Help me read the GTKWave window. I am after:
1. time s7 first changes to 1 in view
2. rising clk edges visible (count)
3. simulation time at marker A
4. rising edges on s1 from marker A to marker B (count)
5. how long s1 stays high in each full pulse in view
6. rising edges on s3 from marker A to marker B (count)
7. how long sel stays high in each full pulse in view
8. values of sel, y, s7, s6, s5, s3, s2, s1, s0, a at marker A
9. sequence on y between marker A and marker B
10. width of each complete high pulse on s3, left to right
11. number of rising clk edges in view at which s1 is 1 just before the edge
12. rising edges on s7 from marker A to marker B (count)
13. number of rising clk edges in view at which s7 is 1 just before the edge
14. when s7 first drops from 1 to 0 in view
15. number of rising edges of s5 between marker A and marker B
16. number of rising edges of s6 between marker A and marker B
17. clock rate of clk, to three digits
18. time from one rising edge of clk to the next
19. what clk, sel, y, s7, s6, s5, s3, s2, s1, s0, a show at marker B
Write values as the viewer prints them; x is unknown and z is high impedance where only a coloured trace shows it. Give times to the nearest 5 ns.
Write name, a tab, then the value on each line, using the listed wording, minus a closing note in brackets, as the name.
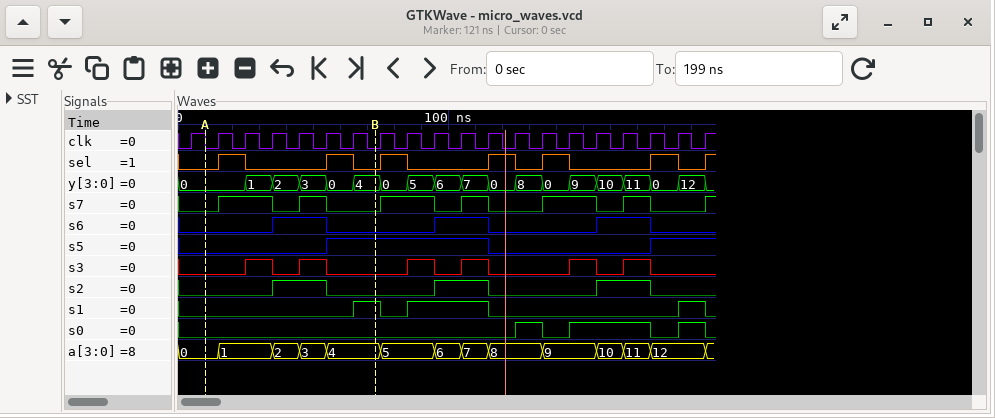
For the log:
time s7 first changes to 1 in view	15 ns
rising clk edges visible	20
simulation time at marker A	10 ns
rising edges on s1 from marker A to marker B	1
how long s1 stays high in each full pulse in view	10 ns, 30 ns, 10 ns
rising edges on s3 from marker A to marker B	2
how long sel stays high in each full pulse in view	10 ns, 10 ns, 10 ns, 10 ns, 10 ns, 10 ns
values of sel, y, s7, s6, s5, s3, s2, s1, s0, a at marker A	sel=0, y=0, s7=0, s6=0, s5=0, s3=0, s2=0, s1=0, s0=0, a=0
sequence on y between marker A and marker B	0, 1, 2, 3, 0, 4
width of each complete high pulse on s3, left to right	10 ns, 10 ns, 10 ns, 10 ns, 10 ns, 10 ns
number of rising clk edges in view at which s1 is 1 just before the edge	5
rising edges on s7 from marker A to marker B	2
number of rising clk edges in view at which s7 is 1 just before the edge	9
when s7 first drops from 1 to 0 in view	35 ns
number of rising edges of s5 between marker A and marker B	1
number of rising edges of s6 between marker A and marker B	1
clock rate of clk, to three digits	100 MHz
time from one rising edge of clk to the next	10 ns
what clk, sel, y, s7, s6, s5, s3, s2, s1, s0, a show at marker B	clk=0, sel=0, y=4, s7=0, s6=0, s5=1, s3=0, s2=0, s1=1, s0=0, a=4
